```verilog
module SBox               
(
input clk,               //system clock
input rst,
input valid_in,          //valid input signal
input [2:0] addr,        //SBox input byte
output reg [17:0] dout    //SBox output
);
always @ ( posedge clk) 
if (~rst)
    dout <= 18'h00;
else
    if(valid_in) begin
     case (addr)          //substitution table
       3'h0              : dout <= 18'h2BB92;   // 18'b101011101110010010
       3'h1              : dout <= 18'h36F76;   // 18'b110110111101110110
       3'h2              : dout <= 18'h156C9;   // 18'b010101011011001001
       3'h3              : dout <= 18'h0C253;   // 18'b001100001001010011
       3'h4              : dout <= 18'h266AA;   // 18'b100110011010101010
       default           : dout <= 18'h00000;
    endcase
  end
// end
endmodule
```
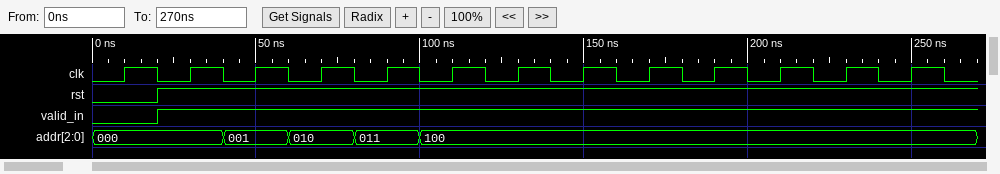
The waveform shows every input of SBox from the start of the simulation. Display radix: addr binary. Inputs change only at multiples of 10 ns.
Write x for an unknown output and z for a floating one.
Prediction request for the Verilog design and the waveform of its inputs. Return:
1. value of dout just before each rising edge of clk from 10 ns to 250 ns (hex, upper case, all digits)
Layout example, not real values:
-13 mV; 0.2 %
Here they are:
x, 00000, 2BB92, 36F76, 156C9, 0C253, 266AA, 266AA, 266AA, 266AA, 266AA, 266AA, 266AA
